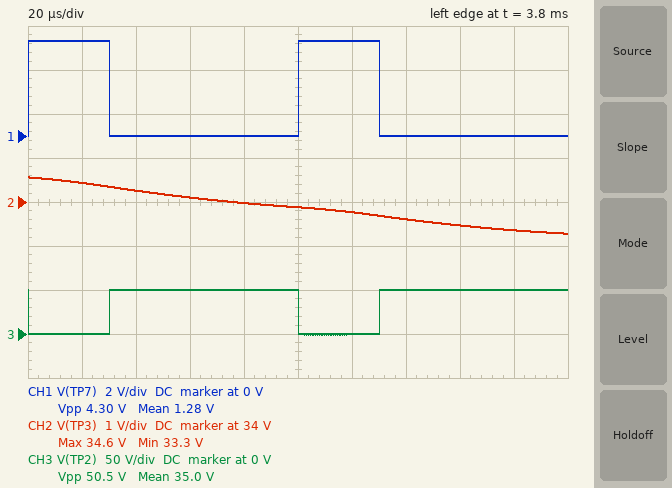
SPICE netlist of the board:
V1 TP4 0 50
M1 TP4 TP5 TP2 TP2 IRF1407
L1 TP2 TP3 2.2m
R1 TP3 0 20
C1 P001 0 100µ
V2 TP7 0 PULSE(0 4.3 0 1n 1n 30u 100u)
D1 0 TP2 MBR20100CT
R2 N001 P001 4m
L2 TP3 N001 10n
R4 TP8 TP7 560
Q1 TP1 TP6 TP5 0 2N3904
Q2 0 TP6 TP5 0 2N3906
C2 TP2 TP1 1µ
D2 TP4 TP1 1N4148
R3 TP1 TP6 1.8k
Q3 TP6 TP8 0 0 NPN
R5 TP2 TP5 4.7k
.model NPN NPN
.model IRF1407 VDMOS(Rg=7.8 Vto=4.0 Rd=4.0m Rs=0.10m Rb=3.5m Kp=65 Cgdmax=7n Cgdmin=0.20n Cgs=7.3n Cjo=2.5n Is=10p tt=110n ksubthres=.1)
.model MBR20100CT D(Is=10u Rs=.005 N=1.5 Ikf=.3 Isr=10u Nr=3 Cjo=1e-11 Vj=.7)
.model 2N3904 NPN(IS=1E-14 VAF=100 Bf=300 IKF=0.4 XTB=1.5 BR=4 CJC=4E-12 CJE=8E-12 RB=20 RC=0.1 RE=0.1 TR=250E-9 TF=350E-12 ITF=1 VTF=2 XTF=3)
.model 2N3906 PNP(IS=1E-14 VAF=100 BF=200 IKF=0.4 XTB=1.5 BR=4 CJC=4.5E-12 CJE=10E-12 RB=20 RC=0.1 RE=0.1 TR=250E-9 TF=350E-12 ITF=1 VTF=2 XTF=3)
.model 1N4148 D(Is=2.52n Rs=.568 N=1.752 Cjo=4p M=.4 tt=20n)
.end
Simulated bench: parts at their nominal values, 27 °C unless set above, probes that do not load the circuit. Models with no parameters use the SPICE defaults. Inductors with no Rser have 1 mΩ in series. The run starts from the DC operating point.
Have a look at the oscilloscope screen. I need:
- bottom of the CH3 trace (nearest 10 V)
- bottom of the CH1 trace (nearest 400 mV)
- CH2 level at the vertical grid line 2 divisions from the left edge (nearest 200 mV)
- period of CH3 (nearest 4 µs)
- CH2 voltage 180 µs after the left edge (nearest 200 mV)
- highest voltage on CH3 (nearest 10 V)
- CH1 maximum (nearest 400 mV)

0 V
0 V
34.2 V
100 µs
33.4 V
50 V
4.4 V
